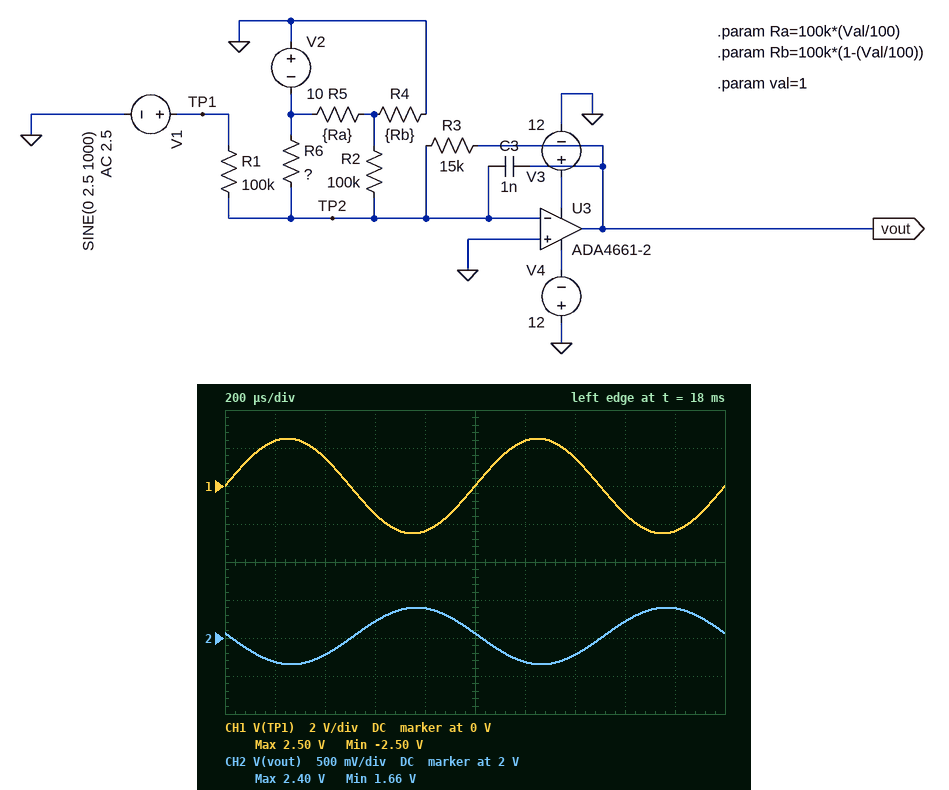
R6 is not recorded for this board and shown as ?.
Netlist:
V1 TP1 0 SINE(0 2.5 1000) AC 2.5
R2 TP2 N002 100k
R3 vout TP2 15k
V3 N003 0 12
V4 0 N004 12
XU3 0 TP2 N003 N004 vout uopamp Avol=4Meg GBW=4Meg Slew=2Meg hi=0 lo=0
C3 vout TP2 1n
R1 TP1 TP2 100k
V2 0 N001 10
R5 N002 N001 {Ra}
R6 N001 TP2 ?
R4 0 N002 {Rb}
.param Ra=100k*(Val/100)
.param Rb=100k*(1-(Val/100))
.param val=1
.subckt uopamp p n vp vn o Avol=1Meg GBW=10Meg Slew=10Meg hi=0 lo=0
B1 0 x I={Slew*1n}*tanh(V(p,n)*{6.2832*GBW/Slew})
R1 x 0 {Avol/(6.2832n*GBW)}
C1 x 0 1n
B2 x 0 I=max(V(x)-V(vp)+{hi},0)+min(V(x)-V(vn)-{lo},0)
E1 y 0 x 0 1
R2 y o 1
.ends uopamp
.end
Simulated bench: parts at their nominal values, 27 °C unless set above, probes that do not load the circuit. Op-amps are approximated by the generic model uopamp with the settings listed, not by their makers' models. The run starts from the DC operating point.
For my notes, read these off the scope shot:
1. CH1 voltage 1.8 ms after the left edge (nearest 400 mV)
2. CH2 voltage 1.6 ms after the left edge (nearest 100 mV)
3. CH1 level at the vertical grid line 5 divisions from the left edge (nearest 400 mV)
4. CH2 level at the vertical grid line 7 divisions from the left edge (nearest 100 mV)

-2.4 V
2.2 V
0 V
1.8 V
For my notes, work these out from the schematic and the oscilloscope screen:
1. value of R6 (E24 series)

270 kΩ
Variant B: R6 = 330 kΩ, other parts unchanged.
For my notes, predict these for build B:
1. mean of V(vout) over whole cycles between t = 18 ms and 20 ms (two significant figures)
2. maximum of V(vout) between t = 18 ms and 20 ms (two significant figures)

1.9 V
2.3 V
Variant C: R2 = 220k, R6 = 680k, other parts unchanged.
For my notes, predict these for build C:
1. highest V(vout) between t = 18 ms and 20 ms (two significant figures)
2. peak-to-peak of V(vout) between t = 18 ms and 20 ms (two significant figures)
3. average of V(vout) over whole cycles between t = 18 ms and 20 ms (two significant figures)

1.3 V
750 mV
890 mV
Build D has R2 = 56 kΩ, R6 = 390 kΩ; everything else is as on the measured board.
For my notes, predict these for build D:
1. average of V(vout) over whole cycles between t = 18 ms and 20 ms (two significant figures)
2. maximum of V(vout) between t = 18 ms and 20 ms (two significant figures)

3.0 V
3.4 V
